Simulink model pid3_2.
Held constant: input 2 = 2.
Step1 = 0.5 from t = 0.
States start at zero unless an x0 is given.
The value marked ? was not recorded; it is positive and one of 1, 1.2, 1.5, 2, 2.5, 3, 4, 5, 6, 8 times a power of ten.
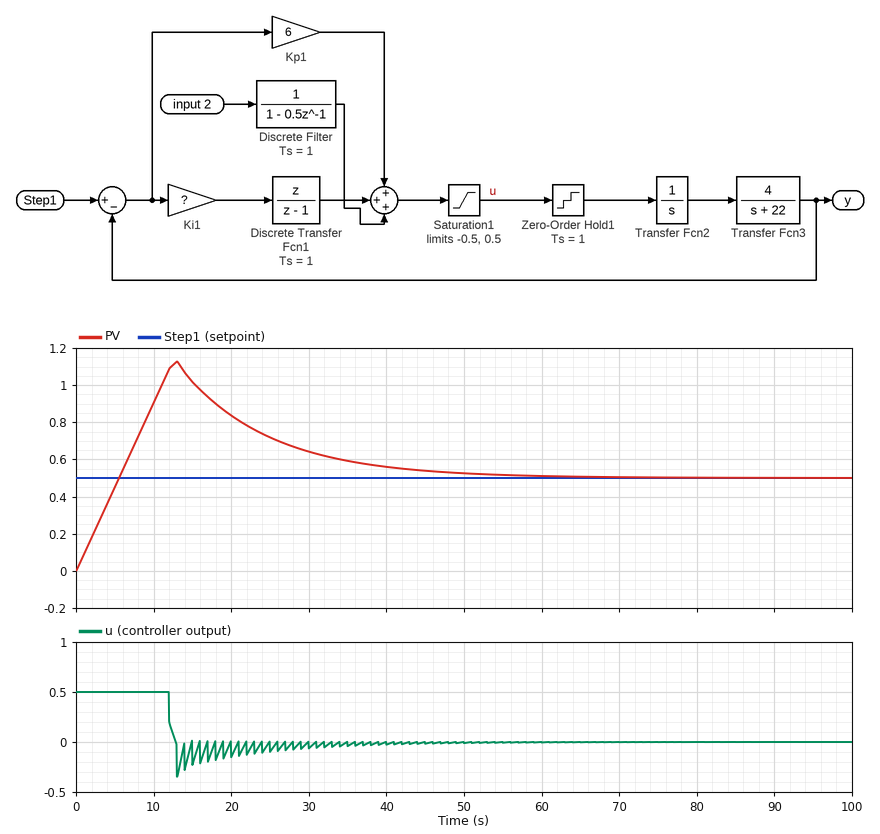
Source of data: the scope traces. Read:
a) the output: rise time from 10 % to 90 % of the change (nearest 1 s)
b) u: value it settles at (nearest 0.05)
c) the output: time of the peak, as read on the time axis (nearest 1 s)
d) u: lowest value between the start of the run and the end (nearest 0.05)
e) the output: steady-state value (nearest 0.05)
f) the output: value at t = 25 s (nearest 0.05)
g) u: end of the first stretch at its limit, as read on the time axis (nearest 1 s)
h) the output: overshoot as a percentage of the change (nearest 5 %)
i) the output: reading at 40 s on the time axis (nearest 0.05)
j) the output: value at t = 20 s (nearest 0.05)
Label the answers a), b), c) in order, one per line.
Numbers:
a) 4 s
b) 0.00
c) 13 s
d) -0.35
e) 0.50
f) 0.70
g) 12 s
h) 125 %
i) 0.55
j) 0.85
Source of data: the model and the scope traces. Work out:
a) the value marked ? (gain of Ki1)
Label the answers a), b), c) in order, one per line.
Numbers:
a) 0.5
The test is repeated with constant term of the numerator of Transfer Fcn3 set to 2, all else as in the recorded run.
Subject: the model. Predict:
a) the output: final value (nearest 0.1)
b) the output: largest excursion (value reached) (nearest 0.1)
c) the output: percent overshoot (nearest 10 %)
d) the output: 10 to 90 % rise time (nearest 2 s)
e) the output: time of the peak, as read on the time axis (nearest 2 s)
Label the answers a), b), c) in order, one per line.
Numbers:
a) 0.5
b) 1.1
c) 120 %
d) 8 s
e) 24 s
